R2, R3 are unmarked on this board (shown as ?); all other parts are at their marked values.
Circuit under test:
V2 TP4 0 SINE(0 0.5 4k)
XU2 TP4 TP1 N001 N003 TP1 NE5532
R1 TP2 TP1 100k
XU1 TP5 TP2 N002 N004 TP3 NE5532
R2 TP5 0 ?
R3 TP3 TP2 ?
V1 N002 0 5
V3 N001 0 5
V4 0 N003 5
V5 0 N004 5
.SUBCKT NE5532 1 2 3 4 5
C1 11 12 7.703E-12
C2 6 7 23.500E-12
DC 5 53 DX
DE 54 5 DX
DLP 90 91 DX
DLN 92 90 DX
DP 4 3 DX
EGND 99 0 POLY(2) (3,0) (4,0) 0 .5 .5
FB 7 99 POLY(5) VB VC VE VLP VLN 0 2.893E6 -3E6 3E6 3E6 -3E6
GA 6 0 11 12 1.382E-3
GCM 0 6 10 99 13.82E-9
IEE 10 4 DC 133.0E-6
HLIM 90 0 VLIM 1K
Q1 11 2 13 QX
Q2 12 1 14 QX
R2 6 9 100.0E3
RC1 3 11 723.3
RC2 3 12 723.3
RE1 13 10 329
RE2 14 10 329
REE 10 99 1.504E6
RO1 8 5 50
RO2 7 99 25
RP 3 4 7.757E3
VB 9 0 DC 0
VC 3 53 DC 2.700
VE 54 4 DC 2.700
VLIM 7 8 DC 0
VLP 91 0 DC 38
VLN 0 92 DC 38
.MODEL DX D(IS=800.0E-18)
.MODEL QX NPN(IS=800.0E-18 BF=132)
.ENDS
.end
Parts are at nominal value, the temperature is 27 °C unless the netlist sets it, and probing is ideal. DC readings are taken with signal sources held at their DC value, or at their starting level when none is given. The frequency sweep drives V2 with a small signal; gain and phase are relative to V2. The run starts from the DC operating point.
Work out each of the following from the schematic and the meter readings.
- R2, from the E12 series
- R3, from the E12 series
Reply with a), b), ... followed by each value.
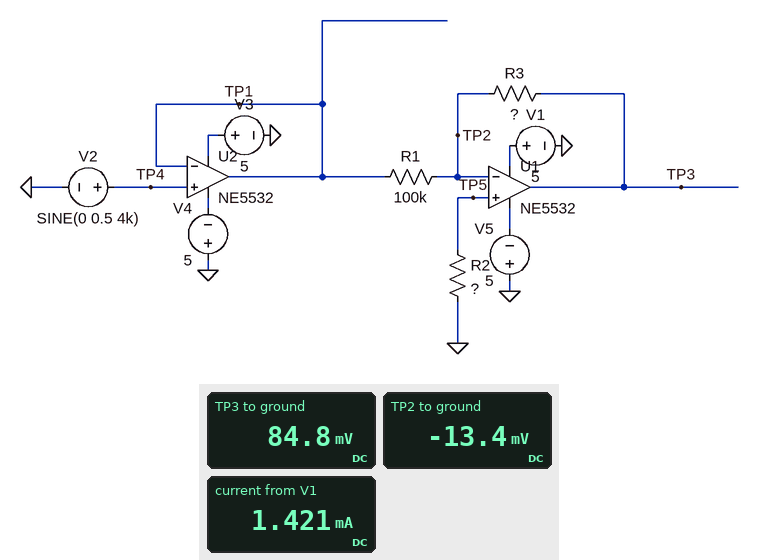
a) 27 kΩ
b) 270 kΩ
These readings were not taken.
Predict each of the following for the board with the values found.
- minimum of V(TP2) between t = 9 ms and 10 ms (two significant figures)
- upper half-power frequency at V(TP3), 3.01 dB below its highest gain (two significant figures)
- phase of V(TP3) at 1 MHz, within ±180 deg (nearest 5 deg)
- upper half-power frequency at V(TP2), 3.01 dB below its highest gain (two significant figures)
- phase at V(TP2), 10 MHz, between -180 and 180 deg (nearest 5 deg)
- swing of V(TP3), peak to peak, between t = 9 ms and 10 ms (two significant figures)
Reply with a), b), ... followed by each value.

a) -14 mV
b) 1.9 MHz
c) 140 deg
d) 13 MHz
e) -70 deg
f) 2.7 V
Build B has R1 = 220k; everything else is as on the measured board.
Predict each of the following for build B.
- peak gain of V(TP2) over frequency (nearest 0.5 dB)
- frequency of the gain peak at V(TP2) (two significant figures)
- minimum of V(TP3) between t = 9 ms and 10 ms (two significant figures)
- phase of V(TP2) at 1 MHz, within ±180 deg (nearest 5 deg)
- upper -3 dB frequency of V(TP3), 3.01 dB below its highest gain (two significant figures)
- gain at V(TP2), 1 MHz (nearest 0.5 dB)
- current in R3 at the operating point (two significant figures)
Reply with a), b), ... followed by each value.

a) -8.0 dB
b) 6.8 MHz
c) -510 mV
d) 65 deg
e) 2.9 MHz
f) -17.0 dB
g) 440 nA
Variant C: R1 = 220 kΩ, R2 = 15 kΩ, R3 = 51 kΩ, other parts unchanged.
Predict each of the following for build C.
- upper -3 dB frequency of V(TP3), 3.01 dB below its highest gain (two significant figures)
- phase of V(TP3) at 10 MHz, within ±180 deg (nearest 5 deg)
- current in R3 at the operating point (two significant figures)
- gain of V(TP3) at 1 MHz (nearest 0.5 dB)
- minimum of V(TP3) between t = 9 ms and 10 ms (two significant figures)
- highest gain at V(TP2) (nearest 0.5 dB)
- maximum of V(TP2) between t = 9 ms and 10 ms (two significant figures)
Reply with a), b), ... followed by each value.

a) 8.1 MHz
b) 5 deg
c) 460 nA
d) -12.5 dB
e) -100 mV
f) -15.0 dB
g) -7.4 mV
